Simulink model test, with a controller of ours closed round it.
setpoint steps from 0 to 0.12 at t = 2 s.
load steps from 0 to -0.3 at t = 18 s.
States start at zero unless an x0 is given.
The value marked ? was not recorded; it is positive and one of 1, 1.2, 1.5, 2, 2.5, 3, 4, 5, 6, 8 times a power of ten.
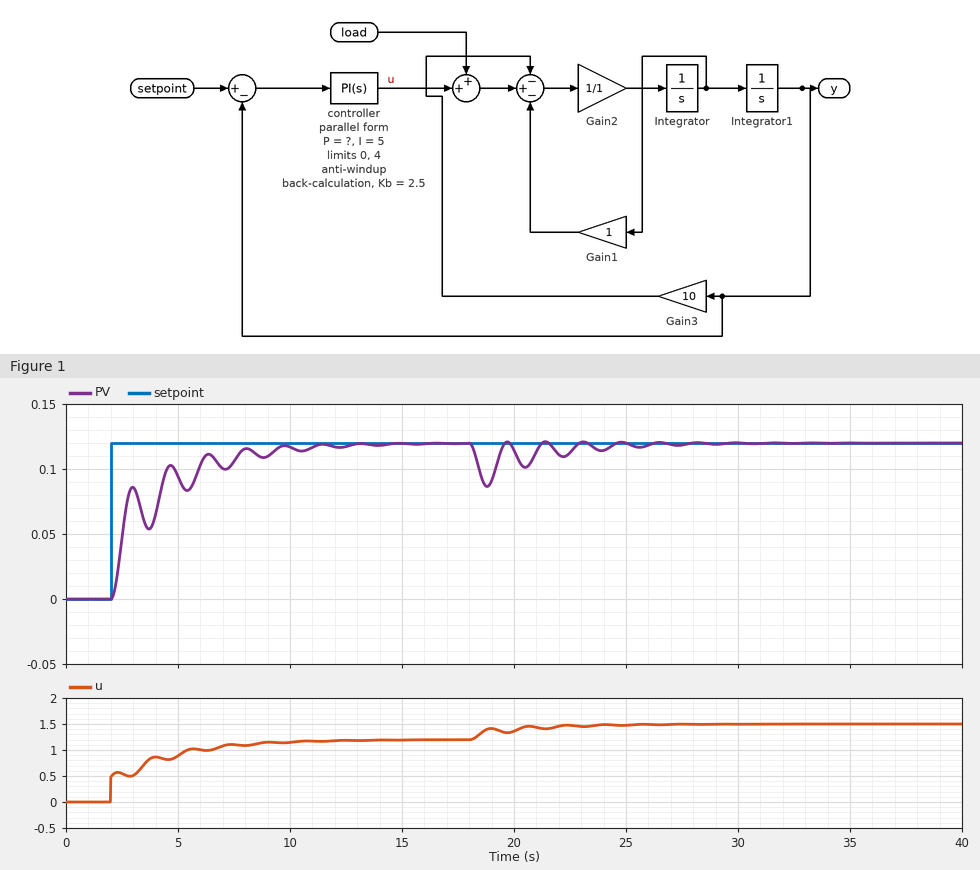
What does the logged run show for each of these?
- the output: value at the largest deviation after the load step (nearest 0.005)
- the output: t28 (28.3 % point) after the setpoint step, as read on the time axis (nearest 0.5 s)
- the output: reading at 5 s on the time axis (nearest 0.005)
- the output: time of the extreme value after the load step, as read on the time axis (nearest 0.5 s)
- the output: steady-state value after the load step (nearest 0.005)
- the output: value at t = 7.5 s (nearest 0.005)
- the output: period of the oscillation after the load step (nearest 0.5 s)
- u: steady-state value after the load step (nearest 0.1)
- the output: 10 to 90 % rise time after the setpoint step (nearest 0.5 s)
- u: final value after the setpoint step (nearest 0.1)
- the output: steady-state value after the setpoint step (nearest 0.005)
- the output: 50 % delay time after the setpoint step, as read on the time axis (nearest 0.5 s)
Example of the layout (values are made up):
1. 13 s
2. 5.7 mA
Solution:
1. 0.085
2. 2.5 s
3. 0.095
4. 19.0 s
5. 0.120
6. 0.105
7. 1.5 s
8. 1.5
9. 4.0 s
10. 1.2
11. 0.120
12. 2.5 s
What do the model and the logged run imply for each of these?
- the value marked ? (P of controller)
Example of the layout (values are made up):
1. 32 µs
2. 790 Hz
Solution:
1. 4
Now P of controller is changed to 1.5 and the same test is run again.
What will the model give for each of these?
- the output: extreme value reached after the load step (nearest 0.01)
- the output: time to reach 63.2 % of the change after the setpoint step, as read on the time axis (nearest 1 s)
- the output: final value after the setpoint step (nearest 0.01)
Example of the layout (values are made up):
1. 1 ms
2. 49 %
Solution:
1. 0.08
2. 4 s
3. 0.12
